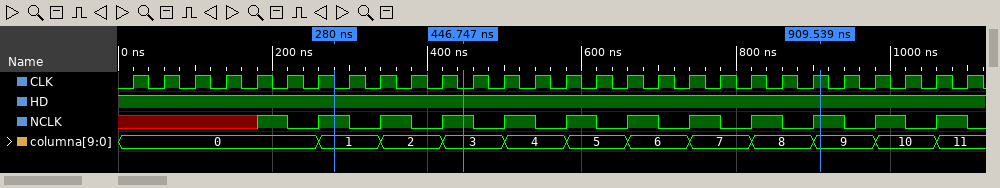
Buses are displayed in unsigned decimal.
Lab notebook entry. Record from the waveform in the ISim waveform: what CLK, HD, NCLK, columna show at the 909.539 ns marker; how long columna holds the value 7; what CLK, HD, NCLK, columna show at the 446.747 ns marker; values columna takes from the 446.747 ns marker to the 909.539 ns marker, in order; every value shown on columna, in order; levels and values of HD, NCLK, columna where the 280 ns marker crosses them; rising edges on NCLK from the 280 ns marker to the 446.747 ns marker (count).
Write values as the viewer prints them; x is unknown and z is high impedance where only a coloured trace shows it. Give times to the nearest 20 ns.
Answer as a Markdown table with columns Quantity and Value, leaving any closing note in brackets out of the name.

| Quantity | Value |
|---|---|
| what CLK, HD, NCLK, columna show at the 909.539 ns marker | CLK=1, HD=1, NCLK=1, columna=9 |
| how long columna holds the value 7 | 80 ns |
| what CLK, HD, NCLK, columna show at the 446.747 ns marker | CLK=0, HD=1, NCLK=1, columna=3 |
| values columna takes from the 446.747 ns marker to the 909.539 ns marker, in order | 3, 4, 5, 6, 7, 8, 9 |
| every value shown on columna, in order | 0, 1, 2, 3, 4, 5, 6, 7, 8, 9, 10, 11 |
| levels and values of HD, NCLK, columna where the 280 ns marker crosses them | HD=1, NCLK=1, columna=1 |
| rising edges on NCLK from the 280 ns marker to the 446.747 ns marker | 2 |
